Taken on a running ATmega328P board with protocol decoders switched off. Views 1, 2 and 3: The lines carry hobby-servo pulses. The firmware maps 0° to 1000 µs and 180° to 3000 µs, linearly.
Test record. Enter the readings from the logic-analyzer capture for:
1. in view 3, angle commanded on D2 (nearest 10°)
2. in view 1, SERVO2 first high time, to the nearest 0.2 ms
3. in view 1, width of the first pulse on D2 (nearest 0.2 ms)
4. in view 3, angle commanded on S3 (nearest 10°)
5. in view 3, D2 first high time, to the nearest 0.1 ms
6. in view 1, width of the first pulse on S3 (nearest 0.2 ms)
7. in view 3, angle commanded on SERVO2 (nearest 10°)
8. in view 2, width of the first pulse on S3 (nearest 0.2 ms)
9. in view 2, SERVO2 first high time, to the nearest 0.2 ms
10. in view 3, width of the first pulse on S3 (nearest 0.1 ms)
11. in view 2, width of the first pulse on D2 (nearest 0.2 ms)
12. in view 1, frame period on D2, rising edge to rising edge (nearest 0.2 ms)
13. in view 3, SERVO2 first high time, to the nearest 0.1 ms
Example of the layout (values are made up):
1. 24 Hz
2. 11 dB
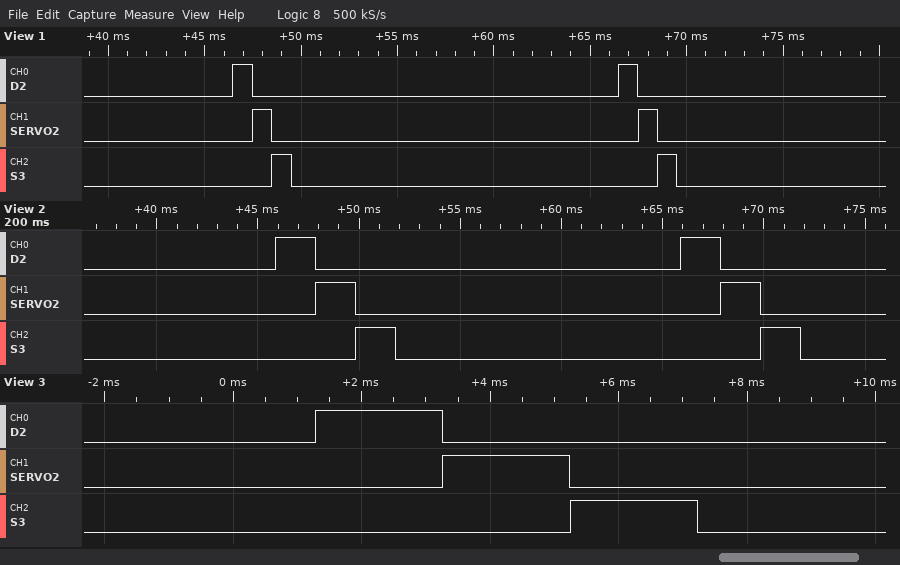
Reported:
1. 90°
2. 1.0 ms
3. 1.0 ms
4. 90°
5. 2.0 ms
6. 1.0 ms
7. 90°
8. 2.0 ms
9. 2.0 ms
10. 2.0 ms
11. 2.0 ms
12. 20.0 ms
13. 2.0 ms
